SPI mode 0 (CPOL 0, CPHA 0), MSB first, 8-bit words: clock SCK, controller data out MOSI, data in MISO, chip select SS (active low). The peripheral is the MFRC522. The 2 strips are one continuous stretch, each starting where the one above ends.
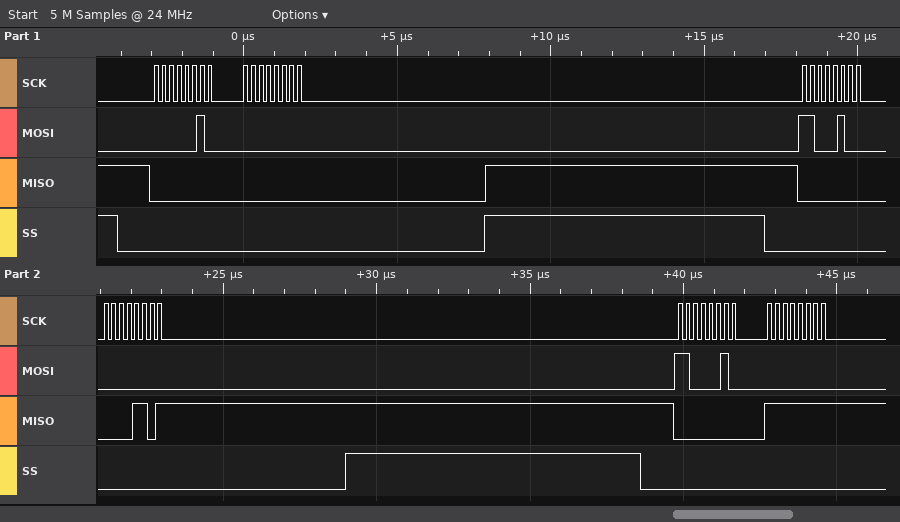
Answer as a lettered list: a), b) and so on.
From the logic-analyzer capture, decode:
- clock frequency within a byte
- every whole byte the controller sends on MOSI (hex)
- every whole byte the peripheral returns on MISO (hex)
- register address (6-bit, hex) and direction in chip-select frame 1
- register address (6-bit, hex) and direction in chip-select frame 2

a) 4 MHz
b) 02 00 C4 00 C2 00
c) 00 00 00 0D 00 FF
d) 0x01 write
e) 0x22 read
